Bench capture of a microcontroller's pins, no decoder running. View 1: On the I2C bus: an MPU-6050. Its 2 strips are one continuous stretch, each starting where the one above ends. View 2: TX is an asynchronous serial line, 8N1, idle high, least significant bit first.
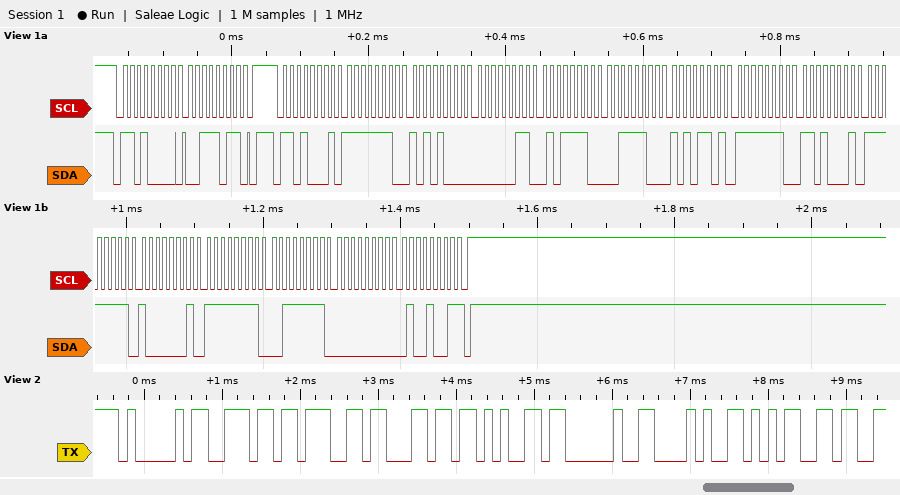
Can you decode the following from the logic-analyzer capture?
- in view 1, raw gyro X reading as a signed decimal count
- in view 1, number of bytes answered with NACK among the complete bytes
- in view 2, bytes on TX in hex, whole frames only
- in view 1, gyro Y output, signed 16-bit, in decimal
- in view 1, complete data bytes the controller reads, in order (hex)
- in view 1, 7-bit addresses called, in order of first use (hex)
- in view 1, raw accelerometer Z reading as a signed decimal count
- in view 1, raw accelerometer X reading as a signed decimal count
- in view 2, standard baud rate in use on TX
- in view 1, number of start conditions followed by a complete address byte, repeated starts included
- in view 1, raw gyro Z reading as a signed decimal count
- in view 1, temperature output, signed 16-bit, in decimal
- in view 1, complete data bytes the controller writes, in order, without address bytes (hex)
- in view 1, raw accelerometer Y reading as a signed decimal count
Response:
-127
1
41 6E 67 6C 65 20 28 35
-193
FE A8 03 5E 3C AD FE D1 FF 81 FF 3F 00 49
0x68
15533
-344
9600 baud
2
73
-303
3B
862
